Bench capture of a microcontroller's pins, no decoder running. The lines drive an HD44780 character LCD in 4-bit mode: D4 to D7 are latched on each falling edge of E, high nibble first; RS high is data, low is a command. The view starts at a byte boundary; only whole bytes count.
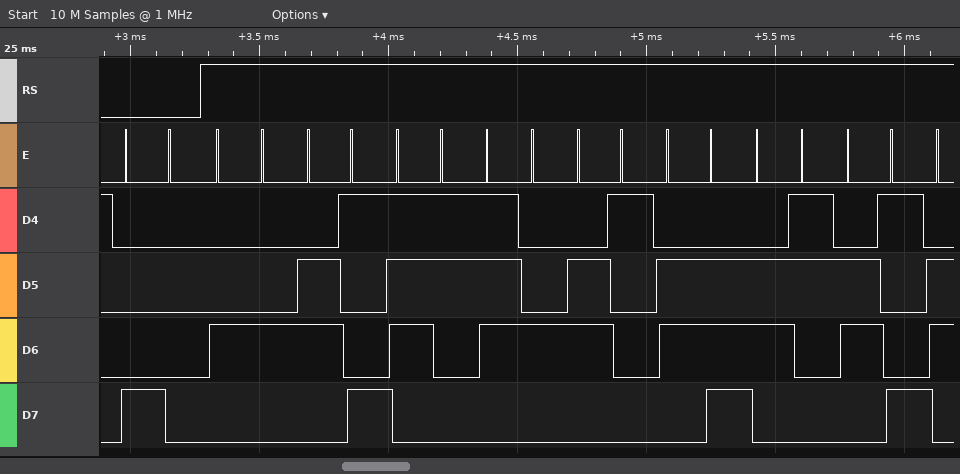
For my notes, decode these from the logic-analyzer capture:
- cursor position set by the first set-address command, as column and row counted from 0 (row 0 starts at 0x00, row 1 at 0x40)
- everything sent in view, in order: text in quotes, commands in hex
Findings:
column 0, row 0
0x80 "Distanci"
